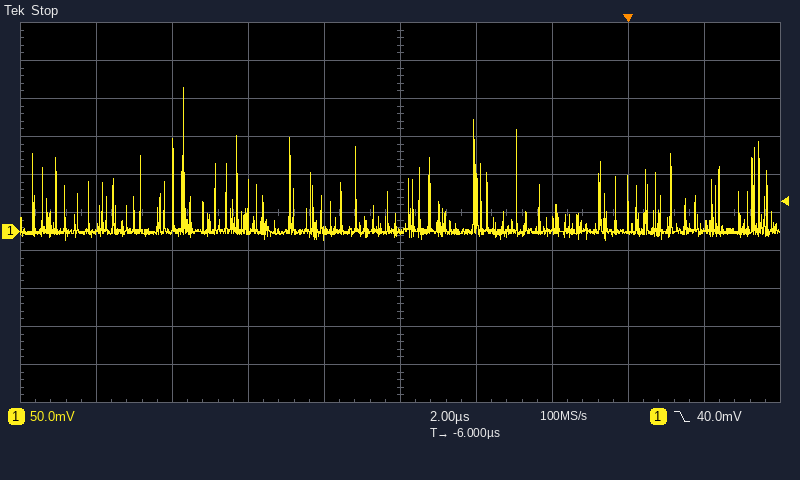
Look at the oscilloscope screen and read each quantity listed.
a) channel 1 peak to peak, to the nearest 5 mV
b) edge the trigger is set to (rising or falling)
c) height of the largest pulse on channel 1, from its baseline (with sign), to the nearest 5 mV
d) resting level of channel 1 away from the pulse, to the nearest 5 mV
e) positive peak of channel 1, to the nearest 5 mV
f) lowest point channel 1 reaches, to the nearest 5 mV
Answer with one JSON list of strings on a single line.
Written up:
["200 mV", "falling", "+190 mV", "0 mV", "190 mV", "-10 mV"]
